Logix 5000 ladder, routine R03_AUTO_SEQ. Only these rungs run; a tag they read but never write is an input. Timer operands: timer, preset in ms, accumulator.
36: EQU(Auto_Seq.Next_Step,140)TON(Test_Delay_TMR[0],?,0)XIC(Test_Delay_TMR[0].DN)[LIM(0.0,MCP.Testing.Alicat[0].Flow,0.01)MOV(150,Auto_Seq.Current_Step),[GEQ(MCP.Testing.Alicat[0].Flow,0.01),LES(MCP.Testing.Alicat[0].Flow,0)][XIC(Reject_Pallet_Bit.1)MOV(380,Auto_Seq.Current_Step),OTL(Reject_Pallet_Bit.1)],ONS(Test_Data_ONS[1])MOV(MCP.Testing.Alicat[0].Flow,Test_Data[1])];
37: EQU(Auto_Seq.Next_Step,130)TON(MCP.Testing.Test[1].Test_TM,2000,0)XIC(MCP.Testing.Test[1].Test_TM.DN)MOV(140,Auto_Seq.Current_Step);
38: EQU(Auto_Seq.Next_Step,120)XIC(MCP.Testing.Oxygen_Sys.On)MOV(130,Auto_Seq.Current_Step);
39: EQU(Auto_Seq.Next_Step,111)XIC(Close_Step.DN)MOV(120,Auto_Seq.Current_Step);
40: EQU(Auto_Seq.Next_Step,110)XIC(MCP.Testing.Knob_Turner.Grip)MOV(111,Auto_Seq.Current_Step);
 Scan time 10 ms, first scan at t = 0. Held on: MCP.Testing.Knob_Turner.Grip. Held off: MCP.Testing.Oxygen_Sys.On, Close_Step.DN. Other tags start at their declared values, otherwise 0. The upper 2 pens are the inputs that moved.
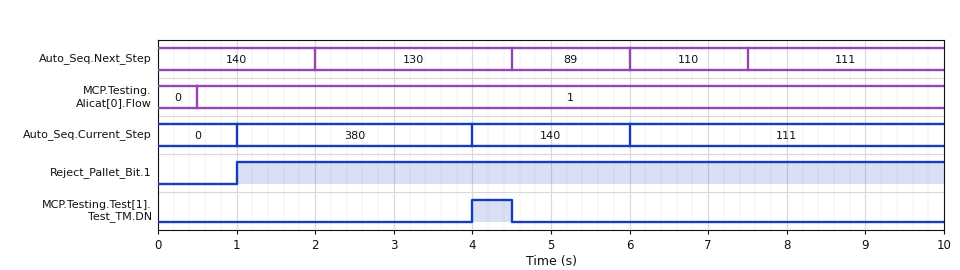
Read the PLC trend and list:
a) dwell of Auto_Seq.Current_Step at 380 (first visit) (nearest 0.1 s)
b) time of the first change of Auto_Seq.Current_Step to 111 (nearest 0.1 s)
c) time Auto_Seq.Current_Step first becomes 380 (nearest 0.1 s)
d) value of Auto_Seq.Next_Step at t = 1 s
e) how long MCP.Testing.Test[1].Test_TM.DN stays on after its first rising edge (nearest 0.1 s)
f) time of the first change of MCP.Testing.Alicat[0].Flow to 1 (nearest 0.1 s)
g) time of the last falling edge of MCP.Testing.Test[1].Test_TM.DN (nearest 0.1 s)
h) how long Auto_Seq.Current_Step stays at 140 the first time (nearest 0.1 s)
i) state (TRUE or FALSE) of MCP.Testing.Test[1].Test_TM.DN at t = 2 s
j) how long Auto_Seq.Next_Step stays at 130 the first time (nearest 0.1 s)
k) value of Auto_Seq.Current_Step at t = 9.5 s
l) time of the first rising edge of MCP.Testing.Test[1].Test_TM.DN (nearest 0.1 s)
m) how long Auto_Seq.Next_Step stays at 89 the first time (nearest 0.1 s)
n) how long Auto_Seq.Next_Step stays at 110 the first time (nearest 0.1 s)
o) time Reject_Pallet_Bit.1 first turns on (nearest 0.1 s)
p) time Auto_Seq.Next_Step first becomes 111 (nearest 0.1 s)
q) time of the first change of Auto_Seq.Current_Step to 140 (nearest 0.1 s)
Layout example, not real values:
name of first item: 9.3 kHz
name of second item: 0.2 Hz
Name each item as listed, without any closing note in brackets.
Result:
dwell of Auto_Seq.Current_Step at 380 (first visit): 3.0 s
time of the first change of Auto_Seq.Current_Step to 111: 6.0 s
time Auto_Seq.Current_Step first becomes 380: 1.0 s
value of Auto_Seq.Next_Step at t = 1 s: 140
how long MCP.Testing.Test[1].Test_TM.DN stays on after its first rising edge: 0.5 s
time of the first change of MCP.Testing.Alicat[0].Flow to 1: 0.5 s
time of the last falling edge of MCP.Testing.Test[1].Test_TM.DN: 4.5 s
how long Auto_Seq.Current_Step stays at 140 the first time: 2.0 s
state (TRUE or FALSE) of MCP.Testing.Test[1].Test_TM.DN at t = 2 s: FALSE
how long Auto_Seq.Next_Step stays at 130 the first time: 2.5 s
value of Auto_Seq.Current_Step at t = 9.5 s: 111
time of the first rising edge of MCP.Testing.Test[1].Test_TM.DN: 4.0 s
how long Auto_Seq.Next_Step stays at 89 the first time: 1.5 s
how long Auto_Seq.Next_Step stays at 110 the first time: 1.5 s
time Reject_Pallet_Bit.1 first turns on: 1.0 s
time Auto_Seq.Next_Step first becomes 111: 7.5 s
time of the first change of Auto_Seq.Current_Step to 140: 4.0 s
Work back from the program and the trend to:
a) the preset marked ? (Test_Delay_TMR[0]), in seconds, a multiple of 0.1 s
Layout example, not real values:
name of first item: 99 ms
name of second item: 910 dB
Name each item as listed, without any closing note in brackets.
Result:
the preset marked ? (Test_Delay_TMR[0]), in seconds, a multiple of 0.1 s: 1.0 s
